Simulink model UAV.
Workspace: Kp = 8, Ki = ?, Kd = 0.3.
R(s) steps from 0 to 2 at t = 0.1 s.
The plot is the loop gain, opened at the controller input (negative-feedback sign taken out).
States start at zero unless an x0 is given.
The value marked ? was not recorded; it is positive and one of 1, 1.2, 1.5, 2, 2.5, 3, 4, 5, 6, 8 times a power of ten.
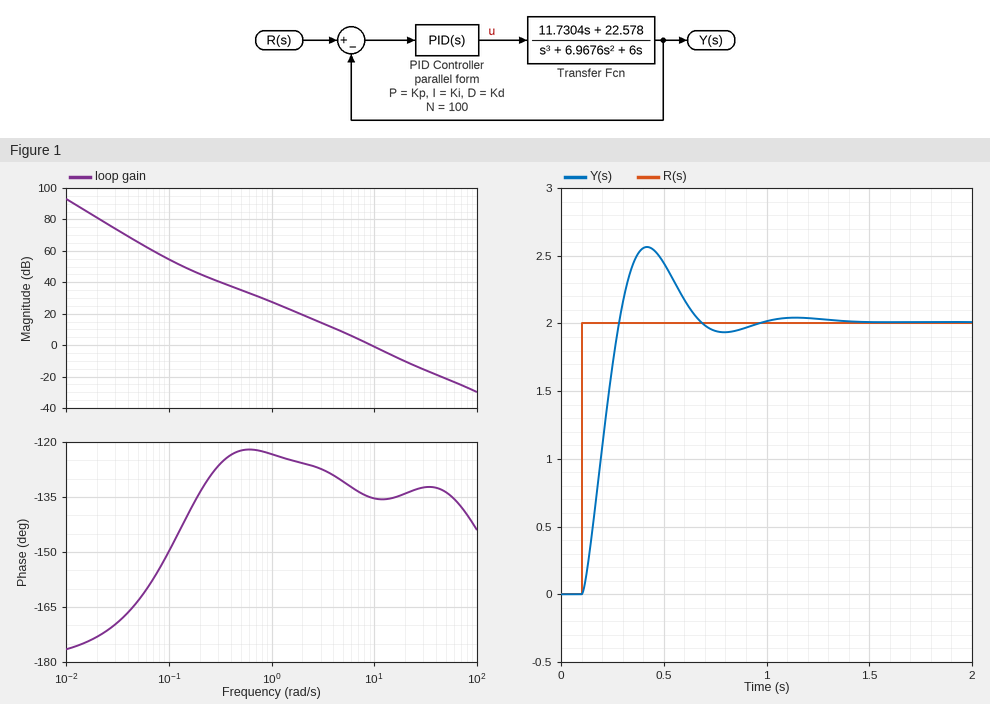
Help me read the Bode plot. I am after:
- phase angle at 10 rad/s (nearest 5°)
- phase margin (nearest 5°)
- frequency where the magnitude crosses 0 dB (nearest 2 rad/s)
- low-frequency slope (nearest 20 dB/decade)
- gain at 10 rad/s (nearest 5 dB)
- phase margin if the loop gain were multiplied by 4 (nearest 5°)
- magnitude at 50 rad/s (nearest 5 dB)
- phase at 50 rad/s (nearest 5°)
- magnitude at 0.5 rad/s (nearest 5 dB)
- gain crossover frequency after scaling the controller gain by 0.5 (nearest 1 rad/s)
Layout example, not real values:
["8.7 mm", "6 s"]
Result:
["-135°", "45°", "10 rad/s", "-40 dB/decade", "0 dB", "45°", "-20 dB", "-135°", "35 dB", "6 rad/s"]
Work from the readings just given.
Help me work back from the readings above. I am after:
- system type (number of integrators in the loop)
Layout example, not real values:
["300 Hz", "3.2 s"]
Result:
["2"]
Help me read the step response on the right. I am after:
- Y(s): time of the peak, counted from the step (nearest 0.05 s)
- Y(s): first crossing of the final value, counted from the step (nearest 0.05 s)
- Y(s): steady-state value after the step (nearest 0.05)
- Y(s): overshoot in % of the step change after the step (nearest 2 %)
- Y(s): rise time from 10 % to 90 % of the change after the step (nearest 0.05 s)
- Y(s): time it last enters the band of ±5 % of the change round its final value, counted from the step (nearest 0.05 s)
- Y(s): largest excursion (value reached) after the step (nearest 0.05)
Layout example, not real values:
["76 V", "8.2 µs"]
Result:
["0.30 s", "0.20 s", "2.00", "28 %", "0.15 s", "0.55 s", "2.55"]
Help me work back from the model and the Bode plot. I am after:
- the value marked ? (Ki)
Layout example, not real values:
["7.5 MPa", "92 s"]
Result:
["1.2"]
